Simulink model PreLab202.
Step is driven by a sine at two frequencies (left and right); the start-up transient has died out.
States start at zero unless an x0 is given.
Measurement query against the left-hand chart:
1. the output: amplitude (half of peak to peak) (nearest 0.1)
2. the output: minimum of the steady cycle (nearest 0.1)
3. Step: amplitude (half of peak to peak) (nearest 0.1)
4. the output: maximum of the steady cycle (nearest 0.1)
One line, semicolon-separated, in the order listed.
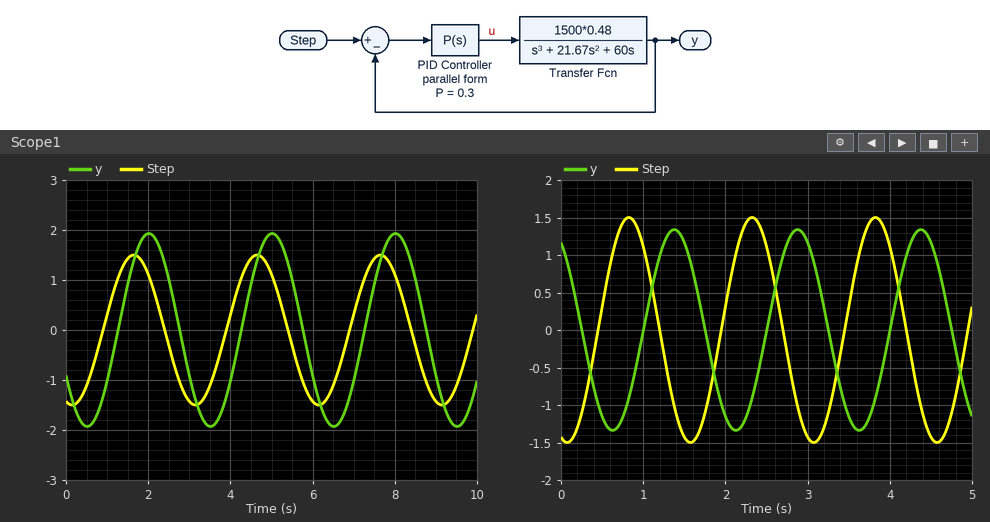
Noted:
1.9; -1.9; 1.5; 1.9
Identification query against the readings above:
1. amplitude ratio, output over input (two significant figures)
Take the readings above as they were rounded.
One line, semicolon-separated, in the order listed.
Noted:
1.3
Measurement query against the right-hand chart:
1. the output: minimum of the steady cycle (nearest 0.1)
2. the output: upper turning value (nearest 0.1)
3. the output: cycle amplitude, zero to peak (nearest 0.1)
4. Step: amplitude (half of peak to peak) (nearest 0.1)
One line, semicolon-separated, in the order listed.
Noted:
-1.3; 1.3; 1.3; 1.5
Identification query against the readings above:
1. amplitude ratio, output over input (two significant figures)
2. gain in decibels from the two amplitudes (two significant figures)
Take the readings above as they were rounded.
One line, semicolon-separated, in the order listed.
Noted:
0.87; -1.2 dB
